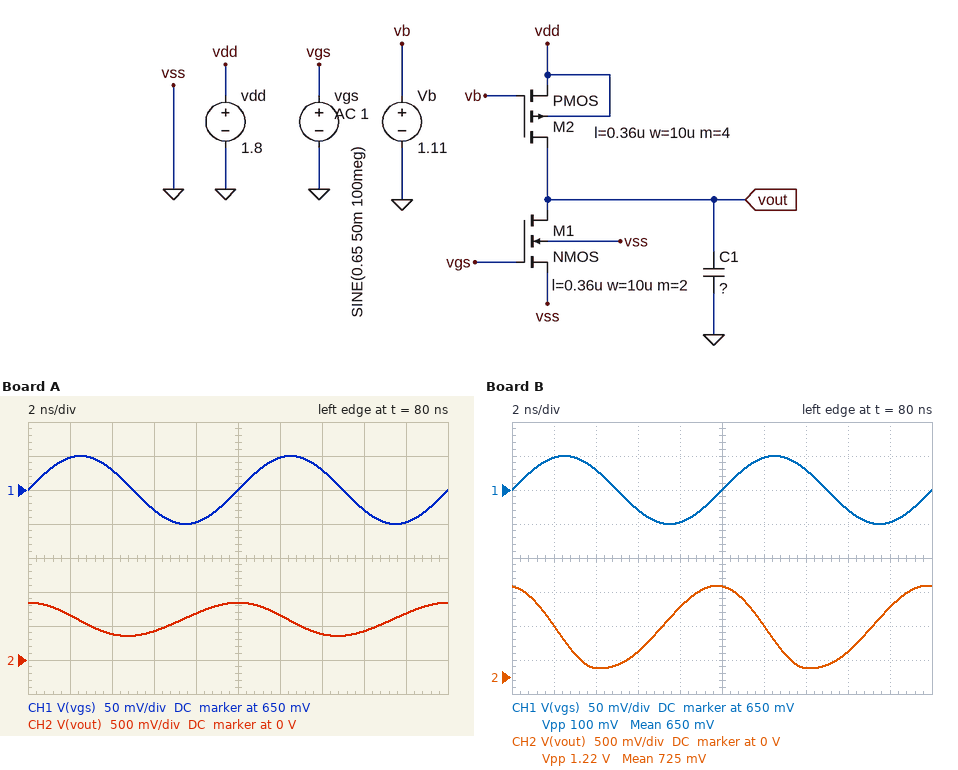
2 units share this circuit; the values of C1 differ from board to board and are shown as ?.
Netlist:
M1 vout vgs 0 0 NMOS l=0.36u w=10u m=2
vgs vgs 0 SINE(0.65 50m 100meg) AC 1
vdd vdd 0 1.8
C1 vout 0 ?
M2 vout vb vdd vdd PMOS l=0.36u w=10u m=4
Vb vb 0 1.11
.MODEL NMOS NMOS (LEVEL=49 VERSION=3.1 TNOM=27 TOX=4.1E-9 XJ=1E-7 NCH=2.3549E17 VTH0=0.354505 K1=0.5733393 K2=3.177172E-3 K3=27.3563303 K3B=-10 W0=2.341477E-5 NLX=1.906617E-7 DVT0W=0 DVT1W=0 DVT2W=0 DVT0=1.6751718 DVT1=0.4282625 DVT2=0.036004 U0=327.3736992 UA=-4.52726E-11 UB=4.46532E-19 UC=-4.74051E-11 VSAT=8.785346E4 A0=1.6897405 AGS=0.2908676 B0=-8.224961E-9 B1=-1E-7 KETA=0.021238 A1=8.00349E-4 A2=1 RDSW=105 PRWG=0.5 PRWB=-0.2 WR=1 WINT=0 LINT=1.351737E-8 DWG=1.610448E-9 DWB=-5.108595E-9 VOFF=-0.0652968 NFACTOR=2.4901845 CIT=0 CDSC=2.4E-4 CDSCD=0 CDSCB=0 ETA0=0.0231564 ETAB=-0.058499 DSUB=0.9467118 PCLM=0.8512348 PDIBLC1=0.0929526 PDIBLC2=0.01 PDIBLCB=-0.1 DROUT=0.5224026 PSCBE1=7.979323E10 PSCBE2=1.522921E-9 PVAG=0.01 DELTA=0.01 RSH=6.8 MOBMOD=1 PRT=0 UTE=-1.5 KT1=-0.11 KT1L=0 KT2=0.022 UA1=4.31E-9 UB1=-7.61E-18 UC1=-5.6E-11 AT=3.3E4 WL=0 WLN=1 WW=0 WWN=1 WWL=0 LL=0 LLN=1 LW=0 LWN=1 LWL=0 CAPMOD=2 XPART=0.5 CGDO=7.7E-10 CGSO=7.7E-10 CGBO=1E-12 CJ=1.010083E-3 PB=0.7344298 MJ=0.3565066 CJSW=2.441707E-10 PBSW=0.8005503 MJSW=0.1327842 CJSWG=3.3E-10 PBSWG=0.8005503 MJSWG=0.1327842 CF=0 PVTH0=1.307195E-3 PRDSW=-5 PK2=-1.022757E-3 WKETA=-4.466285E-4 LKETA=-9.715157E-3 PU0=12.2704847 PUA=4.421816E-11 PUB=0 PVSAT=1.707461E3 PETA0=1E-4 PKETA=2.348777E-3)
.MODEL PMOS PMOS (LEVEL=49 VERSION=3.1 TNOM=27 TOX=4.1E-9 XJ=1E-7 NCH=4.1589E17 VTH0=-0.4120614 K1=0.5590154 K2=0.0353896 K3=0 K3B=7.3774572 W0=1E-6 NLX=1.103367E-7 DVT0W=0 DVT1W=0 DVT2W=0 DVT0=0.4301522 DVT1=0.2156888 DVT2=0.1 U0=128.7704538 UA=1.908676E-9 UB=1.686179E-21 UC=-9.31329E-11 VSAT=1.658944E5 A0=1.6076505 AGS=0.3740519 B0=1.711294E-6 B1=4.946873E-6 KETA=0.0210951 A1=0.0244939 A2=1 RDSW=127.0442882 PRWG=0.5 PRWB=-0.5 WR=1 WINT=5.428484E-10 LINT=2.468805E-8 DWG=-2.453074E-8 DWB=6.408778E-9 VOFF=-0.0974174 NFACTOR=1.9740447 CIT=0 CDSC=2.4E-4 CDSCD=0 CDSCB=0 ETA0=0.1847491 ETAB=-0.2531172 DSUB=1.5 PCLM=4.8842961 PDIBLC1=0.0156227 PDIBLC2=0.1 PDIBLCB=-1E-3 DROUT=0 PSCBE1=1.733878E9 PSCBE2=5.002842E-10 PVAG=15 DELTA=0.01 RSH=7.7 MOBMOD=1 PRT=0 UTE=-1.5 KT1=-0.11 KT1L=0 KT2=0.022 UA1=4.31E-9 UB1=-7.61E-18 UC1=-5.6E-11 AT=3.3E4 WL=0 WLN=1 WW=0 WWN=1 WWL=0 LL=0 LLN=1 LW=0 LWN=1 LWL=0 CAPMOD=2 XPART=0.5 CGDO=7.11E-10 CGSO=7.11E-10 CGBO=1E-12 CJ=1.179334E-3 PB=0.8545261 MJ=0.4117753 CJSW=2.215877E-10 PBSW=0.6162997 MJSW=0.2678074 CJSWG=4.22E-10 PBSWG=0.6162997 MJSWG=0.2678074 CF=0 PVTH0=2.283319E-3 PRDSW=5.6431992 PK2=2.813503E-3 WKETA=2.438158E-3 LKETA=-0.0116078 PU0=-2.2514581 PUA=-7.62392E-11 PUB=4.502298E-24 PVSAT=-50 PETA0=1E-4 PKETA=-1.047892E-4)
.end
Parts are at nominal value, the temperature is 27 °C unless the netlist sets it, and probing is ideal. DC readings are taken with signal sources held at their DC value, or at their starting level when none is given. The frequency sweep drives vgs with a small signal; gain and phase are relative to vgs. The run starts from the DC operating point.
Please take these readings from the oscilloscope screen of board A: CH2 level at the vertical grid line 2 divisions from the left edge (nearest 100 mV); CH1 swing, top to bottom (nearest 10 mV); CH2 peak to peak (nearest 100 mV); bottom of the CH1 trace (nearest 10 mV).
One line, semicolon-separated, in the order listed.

400 mV; 100 mV; 500 mV; 600 mV
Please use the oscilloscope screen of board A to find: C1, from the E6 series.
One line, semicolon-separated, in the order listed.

680 fF
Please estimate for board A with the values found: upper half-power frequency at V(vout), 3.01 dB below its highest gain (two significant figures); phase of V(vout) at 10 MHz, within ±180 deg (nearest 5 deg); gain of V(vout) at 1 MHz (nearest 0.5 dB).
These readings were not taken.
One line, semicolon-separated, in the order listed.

8.2 MHz; 130 deg; 35.5 dB
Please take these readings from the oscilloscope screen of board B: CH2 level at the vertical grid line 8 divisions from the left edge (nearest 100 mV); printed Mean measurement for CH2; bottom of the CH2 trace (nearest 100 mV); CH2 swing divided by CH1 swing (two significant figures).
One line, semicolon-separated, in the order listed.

400 mV; 725 mV; 100 mV; 12
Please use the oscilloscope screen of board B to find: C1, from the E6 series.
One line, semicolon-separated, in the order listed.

220 fF
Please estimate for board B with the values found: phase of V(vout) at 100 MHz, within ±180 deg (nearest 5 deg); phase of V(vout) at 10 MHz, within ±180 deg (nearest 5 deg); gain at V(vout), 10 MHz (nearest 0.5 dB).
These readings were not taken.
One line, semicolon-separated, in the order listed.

100 deg; 155 deg; 35.0 dB
